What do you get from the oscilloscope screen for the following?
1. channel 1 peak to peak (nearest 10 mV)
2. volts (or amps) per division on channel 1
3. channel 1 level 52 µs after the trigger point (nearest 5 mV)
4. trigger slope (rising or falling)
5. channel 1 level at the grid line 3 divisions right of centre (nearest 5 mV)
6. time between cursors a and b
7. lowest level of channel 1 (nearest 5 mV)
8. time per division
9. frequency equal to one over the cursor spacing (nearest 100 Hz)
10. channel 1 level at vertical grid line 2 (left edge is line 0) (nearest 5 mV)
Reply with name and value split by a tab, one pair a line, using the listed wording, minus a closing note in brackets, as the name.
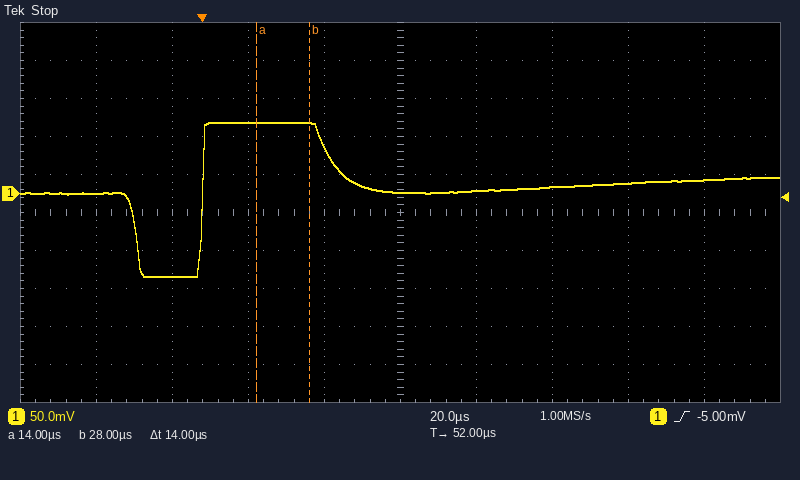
channel 1 peak to peak	200 mV
volts (or amps) per division on channel 1	50 mV
channel 1 level 52 µs after the trigger point	0 mV
trigger slope	rising
channel 1 level at the grid line 3 divisions right of centre	15 mV
time between cursors a and b	14 µs
lowest level of channel 1	-110 mV
time per division	20 µs
frequency equal to one over the cursor spacing	71.4 kHz
channel 1 level at vertical grid line 2 (left edge is line 0)	-110 mV
